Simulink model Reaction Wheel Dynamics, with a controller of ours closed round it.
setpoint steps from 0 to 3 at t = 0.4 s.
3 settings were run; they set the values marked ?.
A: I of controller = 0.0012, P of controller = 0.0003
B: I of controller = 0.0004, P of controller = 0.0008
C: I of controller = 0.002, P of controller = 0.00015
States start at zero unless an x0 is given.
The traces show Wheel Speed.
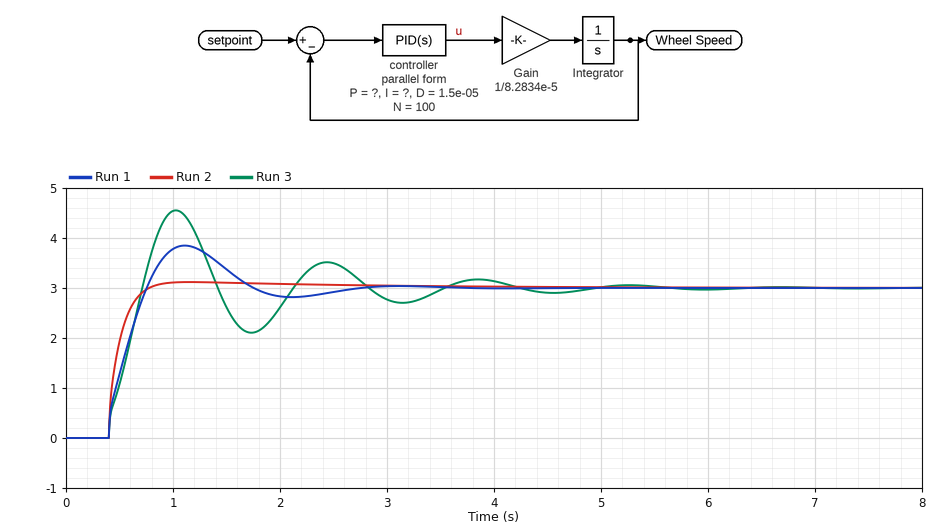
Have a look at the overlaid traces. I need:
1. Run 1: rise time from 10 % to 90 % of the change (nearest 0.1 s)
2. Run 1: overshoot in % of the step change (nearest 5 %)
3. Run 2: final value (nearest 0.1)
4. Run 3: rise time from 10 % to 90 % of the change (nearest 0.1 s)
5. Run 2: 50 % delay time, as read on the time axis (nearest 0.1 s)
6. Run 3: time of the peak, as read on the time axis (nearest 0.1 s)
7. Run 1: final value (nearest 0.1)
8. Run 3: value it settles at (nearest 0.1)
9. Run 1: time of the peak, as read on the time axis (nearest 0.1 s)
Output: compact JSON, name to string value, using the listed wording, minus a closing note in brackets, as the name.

{"Run 1: rise time from 10 % to 90 % of the change": "0.3 s", "Run 1: overshoot in % of the step change": "30 %", "Run 2: final value": "3.0", "Run 3: rise time from 10 % to 90 % of the change": "0.3 s", "Run 2: 50 % delay time, as read on the time axis": "0.5 s", "Run 3: time of the peak, as read on the time axis": "1.0 s", "Run 1: final value": "3.0", "Run 3: value it settles at": "3.0", "Run 1: time of the peak, as read on the time axis": "1.1 s"}
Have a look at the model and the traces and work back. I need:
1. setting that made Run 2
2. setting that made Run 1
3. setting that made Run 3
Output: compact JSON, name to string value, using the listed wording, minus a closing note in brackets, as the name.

{"setting that made Run 2": "B", "setting that made Run 1": "A", "setting that made Run 3": "C"}
